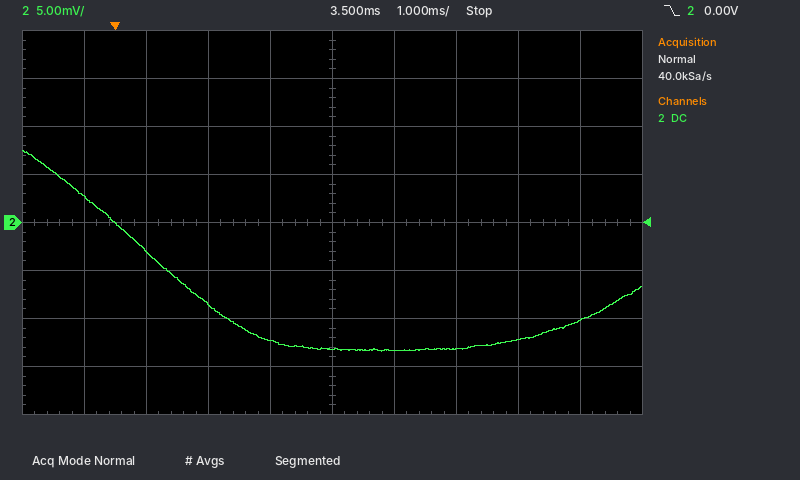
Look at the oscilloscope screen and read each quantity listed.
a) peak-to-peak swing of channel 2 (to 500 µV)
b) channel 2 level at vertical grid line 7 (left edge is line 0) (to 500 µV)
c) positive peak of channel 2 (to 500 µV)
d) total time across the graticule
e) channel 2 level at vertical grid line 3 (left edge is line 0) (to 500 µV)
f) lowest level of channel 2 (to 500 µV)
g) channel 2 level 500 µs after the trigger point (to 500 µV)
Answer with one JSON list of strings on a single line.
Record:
["21.0 mV", "-13.0 mV", "7.5 mV", "10 ms", "-8.5 mV", "-13.5 mV", "-3.0 mV"]
